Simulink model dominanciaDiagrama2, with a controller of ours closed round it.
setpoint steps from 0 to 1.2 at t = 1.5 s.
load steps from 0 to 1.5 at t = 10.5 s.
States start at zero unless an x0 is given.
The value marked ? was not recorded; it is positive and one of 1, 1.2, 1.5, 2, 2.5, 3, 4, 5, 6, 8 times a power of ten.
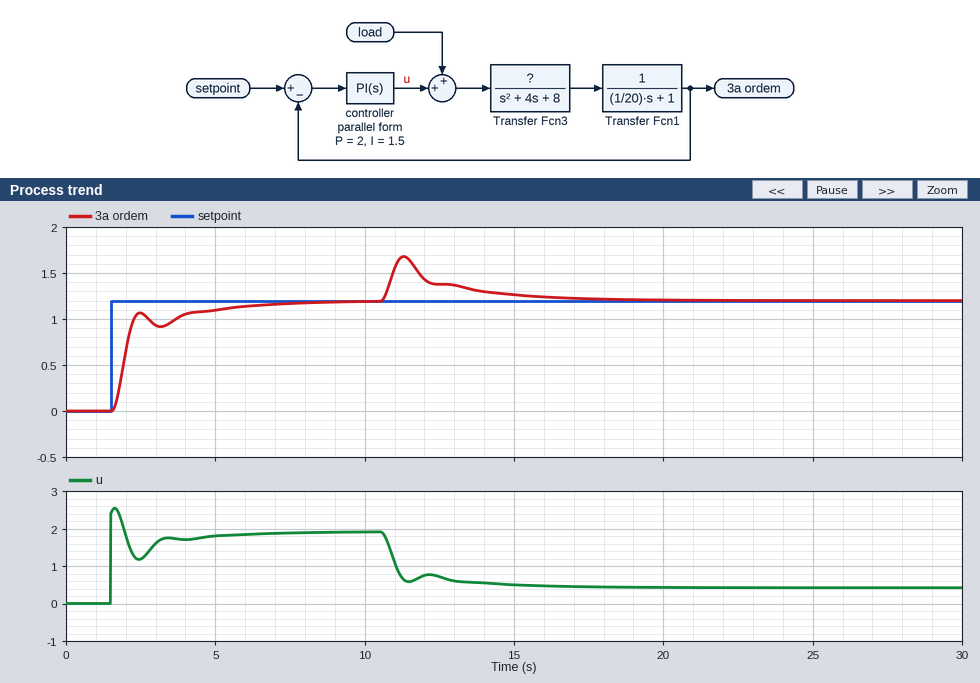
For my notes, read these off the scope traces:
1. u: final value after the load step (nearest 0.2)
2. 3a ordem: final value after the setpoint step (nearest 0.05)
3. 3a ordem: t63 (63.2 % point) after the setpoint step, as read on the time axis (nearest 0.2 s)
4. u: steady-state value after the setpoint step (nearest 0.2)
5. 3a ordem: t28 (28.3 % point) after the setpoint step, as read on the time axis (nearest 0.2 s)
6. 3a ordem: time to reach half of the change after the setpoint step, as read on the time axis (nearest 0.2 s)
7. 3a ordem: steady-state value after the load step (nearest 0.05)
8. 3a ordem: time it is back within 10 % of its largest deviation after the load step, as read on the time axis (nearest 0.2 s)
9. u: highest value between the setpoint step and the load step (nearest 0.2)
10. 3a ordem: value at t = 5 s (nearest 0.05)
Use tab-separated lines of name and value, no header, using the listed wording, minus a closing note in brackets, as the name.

u: final value after the load step	0.4
3a ordem: final value after the setpoint step	1.20
3a ordem: t63 (63.2 % point) after the setpoint step, as read on the time axis	2.0 s
u: steady-state value after the setpoint step	2.0
3a ordem: t28 (28.3 % point) after the setpoint step, as read on the time axis	1.8 s
3a ordem: time to reach half of the change after the setpoint step, as read on the time axis	2.0 s
3a ordem: steady-state value after the load step	1.20
3a ordem: time it is back within 10 % of its largest deviation after the load step, as read on the time axis	15.6 s
u: highest value between the setpoint step and the load step	2.6
3a ordem: value at t = 5 s	1.10
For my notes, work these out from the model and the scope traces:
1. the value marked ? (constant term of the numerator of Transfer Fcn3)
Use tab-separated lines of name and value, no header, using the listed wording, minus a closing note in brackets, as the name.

the value marked ?	5
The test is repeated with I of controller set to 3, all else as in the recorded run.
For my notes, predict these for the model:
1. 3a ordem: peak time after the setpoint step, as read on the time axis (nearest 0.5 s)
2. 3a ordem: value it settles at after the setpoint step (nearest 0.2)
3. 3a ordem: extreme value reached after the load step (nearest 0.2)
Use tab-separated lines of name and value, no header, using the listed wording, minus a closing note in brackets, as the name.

3a ordem: peak time after the setpoint step, as read on the time axis	2.5 s
3a ordem: value it settles at after the setpoint step	1.2
3a ordem: extreme value reached after the load step	1.6
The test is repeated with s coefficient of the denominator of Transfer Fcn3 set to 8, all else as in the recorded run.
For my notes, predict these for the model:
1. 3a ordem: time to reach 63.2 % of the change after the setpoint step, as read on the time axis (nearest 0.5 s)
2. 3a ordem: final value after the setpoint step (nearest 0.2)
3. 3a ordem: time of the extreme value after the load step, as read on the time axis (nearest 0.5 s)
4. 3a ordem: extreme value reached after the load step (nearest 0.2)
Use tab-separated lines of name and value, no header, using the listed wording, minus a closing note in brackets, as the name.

3a ordem: time to reach 63.2 % of the change after the setpoint step, as read on the time axis	2.5 s
3a ordem: final value after the setpoint step	1.2
3a ordem: time of the extreme value after the load step, as read on the time axis	11.5 s
3a ordem: extreme value reached after the load step	1.6
